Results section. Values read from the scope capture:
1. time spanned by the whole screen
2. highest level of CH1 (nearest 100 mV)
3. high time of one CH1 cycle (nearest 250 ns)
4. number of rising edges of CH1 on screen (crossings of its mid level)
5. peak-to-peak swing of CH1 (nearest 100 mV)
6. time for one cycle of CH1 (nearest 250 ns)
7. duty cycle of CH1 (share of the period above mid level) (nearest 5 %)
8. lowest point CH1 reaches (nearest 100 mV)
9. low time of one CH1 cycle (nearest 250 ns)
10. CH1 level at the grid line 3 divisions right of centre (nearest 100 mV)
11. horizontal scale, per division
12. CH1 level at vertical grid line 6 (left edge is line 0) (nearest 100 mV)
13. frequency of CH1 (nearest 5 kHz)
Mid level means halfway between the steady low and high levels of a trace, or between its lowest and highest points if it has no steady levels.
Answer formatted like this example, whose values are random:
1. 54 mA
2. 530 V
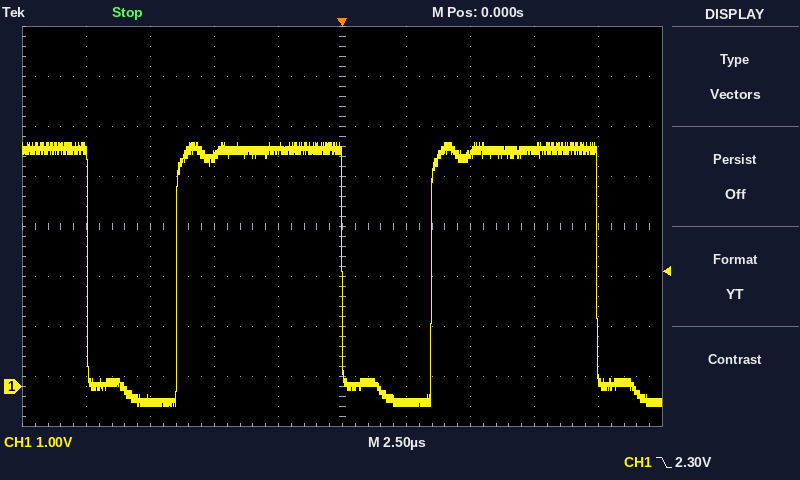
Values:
1. 25 µs
2. 4.9 V
3. 6.50 µs
4. 2
5. 5.3 V
6. 10.00 µs
7. 65 %
8. -400 mV
9. 3.50 µs
10. 4.7 V
11. 2.5 µs
12. -300 mV
13. 100 kHz
